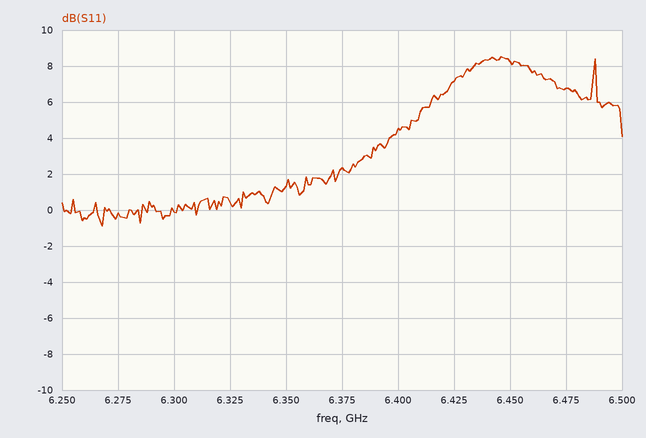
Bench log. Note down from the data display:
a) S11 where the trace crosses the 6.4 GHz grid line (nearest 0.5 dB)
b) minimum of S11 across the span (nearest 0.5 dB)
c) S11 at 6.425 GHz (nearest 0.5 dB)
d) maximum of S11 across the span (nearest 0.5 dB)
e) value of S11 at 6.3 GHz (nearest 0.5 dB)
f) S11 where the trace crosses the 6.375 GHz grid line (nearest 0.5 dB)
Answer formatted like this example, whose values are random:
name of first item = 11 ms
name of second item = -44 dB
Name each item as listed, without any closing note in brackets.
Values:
S11 where the trace crosses the 6.4 GHz grid line = 4.5 dB
minimum of S11 across the span = -1.0 dB
S11 at 6.425 GHz = 7.0 dB
maximum of S11 across the span = 8.5 dB
value of S11 at 6.3 GHz = 0.0 dB
S11 where the trace crosses the 6.375 GHz grid line = 2.5 dB
